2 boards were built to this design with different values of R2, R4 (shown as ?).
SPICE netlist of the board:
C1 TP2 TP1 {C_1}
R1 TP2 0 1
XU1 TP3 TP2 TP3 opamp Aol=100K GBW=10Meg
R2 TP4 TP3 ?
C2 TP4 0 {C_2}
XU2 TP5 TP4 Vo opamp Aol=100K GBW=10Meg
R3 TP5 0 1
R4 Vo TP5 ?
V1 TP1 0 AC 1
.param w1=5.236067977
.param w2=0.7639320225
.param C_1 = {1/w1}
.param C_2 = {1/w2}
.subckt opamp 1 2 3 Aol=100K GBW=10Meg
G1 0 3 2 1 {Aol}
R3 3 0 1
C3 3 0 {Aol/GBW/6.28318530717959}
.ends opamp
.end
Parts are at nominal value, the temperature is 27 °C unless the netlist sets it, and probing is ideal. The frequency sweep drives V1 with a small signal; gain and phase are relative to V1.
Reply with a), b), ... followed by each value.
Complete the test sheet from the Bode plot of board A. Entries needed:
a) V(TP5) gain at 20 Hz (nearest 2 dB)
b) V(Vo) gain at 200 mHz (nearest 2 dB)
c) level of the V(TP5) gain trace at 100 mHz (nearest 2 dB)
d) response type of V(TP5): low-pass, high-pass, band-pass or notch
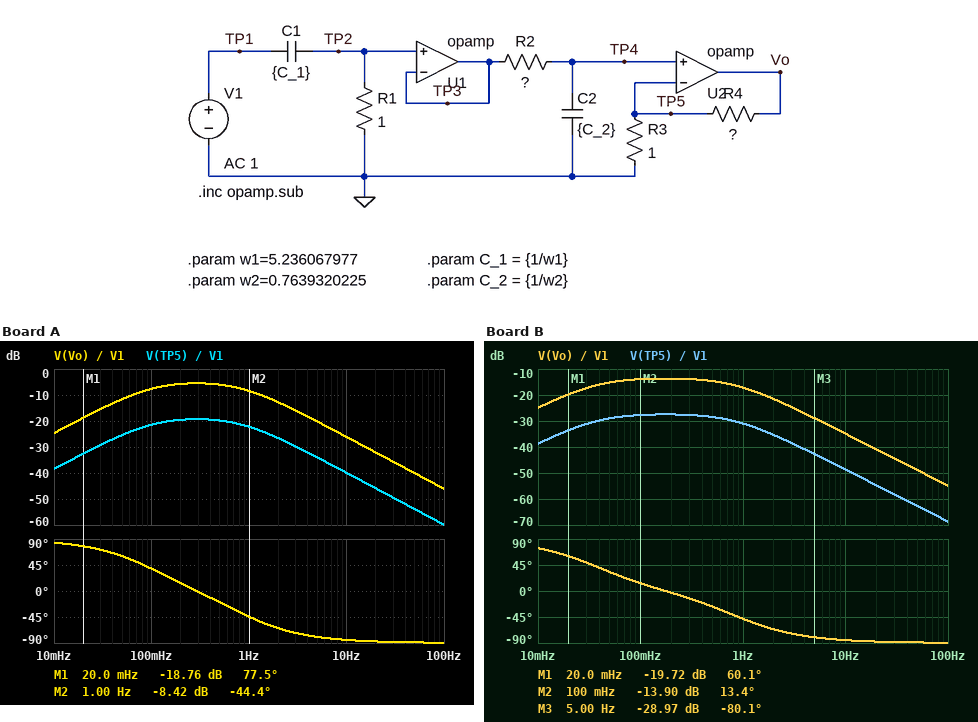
a) -46 dB
b) -6 dB
c) -22 dB
d) band-pass
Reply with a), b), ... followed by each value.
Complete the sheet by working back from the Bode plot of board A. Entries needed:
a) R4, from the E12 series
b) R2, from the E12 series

a) 3.9 Ω
b) 1.2 Ω
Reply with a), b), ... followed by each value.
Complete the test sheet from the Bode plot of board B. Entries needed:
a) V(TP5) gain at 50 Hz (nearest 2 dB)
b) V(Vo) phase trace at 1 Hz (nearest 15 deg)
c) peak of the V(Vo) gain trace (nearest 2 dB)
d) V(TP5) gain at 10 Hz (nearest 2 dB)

a) -62 dB
b) -45 deg
c) -14 dB
d) -48 dB
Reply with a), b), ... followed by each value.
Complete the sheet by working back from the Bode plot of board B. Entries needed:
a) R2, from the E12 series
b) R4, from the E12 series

a) 3.3 Ω
b) 3.9 Ω
